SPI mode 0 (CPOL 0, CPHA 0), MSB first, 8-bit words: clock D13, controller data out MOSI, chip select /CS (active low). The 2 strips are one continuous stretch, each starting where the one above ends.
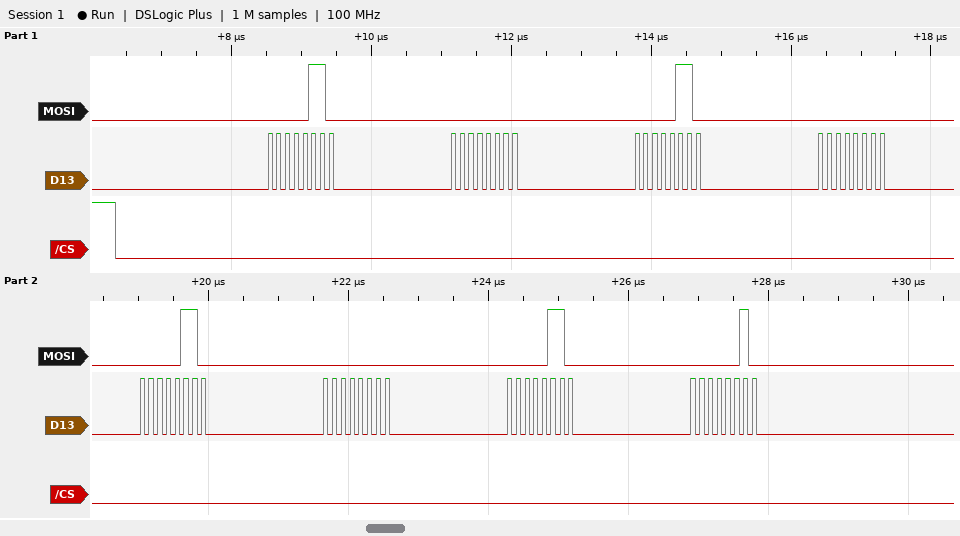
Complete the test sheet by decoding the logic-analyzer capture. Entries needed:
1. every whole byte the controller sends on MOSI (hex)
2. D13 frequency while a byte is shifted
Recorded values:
06 00 06 00 06 00 06 02
8 MHz
